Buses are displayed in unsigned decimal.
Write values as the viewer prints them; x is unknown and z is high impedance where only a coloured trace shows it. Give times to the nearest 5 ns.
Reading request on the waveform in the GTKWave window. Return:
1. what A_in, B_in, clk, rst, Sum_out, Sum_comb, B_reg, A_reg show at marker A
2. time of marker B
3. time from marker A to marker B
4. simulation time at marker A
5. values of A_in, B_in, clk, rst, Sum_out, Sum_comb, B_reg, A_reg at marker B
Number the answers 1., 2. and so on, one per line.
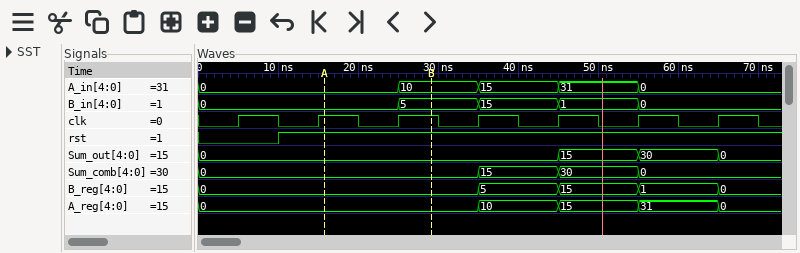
1. A_in=0, B_in=0, clk=1, rst=1, Sum_out=0, Sum_comb=0, B_reg=0, A_reg=0
2. 30 ns
3. 15 ns
4. 15 ns
5. A_in=10, B_in=5, clk=1, rst=1, Sum_out=0, Sum_comb=0, B_reg=0, A_reg=0
